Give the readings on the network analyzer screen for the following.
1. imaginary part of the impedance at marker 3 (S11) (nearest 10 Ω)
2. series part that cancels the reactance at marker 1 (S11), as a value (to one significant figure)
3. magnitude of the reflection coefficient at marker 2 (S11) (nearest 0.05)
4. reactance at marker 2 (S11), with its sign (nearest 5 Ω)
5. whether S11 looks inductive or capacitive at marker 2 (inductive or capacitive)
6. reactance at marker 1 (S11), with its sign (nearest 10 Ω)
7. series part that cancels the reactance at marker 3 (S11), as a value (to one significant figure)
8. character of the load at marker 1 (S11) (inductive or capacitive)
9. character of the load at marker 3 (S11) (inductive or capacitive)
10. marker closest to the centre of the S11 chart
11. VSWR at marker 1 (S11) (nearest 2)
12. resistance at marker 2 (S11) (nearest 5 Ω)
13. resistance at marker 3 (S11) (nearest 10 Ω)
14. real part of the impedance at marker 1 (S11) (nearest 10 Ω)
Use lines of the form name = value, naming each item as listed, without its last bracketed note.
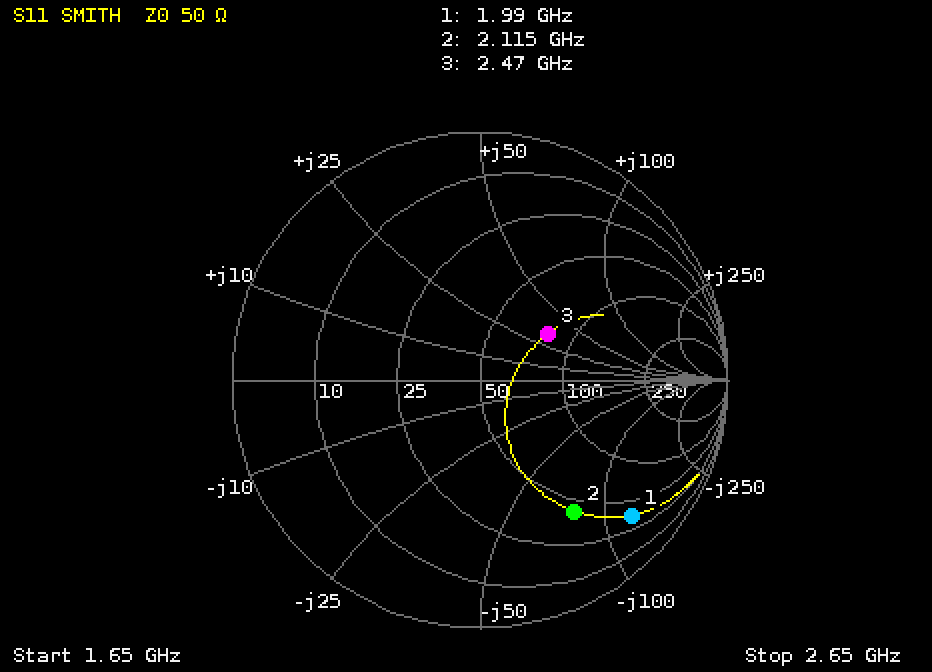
imaginary part of the impedance at marker 3 (S11) = +30 Ω
series part that cancels the reactance at marker 1 (S11), as a value = 10 nH
magnitude of the reflection coefficient at marker 2 (S11) = 0.65
reactance at marker 2 (S11), with its sign = -80 Ω
whether S11 looks inductive or capacitive at marker 2 = capacitive
reactance at marker 1 (S11), with its sign = -120 Ω
series part that cancels the reactance at marker 3 (S11), as a value = 2 pF
character of the load at marker 1 (S11) = capacitive
character of the load at marker 3 (S11) = inductive
marker closest to the centre of the S11 chart = marker 3
VSWR at marker 1 (S11) = 10
resistance at marker 2 (S11) = 45 Ω
resistance at marker 3 (S11) = 80 Ω
real part of the impedance at marker 1 (S11) = 40 Ω
